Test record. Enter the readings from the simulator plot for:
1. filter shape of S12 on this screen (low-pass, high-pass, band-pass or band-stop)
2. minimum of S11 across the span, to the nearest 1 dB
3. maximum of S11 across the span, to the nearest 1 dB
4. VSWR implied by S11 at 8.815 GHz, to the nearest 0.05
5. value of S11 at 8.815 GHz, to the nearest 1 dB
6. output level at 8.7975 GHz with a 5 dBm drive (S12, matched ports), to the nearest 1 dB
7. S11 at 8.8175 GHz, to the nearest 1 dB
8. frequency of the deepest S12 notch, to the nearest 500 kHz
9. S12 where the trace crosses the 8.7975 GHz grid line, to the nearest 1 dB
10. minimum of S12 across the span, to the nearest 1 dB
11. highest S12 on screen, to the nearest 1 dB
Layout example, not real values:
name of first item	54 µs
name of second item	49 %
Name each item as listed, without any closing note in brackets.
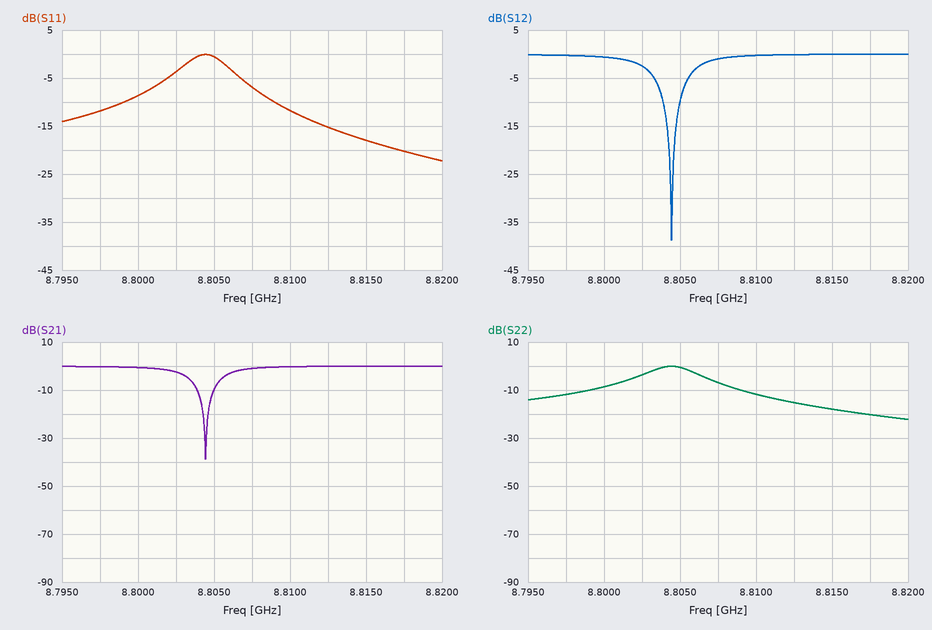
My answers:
filter shape of S12 on this screen	band-stop
minimum of S11 across the span, to the nearest 1 dB	-22 dB
maximum of S11 across the span, to the nearest 1 dB	0 dB
VSWR implied by S11 at 8.815 GHz, to the nearest 0.05	1.30
value of S11 at 8.815 GHz, to the nearest 1 dB	-18 dB
output level at 8.7975 GHz with a 5 dBm drive (S12, matched ports), to the nearest 1 dB	5 dBm
S11 at 8.8175 GHz, to the nearest 1 dB	-20 dB
frequency of the deepest S12 notch, to the nearest 500 kHz	8.8045 GHz
S12 where the trace crosses the 8.7975 GHz grid line, to the nearest 1 dB	0 dB
minimum of S12 across the span, to the nearest 1 dB	-39 dB
highest S12 on screen, to the nearest 1 dB	0 dB
